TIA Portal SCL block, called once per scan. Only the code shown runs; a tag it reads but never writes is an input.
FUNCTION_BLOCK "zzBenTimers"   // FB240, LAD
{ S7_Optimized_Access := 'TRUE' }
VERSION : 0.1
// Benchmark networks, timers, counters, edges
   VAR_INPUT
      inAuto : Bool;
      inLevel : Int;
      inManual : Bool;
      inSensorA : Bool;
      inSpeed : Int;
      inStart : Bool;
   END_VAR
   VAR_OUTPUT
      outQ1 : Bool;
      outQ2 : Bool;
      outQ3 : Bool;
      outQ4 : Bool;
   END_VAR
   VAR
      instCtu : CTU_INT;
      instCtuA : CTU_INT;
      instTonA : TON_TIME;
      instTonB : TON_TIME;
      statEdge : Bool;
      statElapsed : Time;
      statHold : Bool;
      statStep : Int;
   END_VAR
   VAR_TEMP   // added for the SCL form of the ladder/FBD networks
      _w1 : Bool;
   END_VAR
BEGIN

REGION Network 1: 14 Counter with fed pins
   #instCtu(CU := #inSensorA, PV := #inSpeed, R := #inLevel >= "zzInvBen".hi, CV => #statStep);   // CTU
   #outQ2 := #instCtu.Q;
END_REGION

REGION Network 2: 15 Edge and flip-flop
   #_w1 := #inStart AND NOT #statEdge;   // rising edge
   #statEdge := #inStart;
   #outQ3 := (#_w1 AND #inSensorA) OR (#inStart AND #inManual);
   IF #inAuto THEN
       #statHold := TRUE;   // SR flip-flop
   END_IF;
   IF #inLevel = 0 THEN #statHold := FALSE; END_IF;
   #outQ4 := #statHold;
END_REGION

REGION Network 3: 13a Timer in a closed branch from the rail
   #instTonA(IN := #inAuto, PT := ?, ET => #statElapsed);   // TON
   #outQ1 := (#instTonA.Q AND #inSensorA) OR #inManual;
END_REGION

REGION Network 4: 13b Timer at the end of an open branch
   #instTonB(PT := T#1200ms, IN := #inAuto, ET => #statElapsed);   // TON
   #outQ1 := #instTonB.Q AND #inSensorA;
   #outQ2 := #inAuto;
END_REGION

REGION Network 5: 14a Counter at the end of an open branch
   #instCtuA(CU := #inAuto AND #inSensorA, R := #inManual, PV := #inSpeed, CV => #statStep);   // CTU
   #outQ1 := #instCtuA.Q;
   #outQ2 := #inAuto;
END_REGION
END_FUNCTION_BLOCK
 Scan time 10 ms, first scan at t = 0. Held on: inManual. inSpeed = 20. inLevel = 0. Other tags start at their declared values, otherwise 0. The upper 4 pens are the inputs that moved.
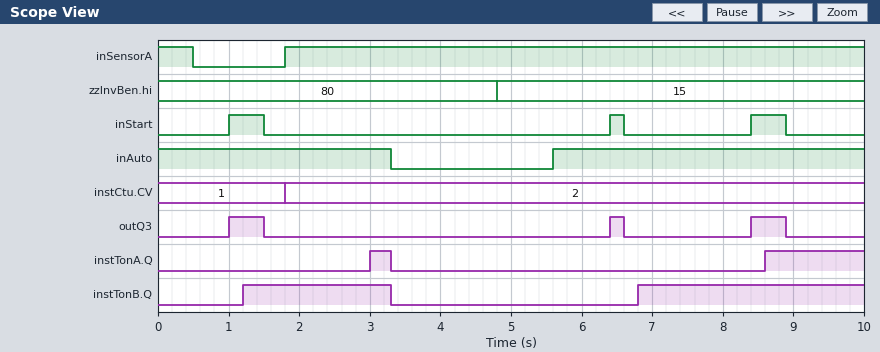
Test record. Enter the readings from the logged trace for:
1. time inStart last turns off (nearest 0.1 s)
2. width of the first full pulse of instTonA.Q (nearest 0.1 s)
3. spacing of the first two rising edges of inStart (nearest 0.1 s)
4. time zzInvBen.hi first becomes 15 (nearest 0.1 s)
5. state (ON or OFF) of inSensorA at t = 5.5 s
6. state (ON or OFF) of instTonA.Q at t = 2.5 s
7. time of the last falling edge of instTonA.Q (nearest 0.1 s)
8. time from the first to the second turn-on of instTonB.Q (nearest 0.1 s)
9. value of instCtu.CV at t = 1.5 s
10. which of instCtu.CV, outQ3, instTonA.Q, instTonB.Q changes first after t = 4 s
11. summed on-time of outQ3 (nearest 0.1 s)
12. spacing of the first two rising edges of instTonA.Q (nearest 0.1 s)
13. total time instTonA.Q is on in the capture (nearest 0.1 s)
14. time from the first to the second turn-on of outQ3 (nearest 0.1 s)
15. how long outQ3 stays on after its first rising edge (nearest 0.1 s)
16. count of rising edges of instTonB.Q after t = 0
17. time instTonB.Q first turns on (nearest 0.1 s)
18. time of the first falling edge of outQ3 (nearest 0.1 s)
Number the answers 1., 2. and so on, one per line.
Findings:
1. 8.9 s
2. 0.3 s
3. 5.4 s
4. 4.8 s
5. ON
6. OFF
7. 3.3 s
8. 5.6 s
9. 1
10. outQ3
11. 1.2 s
12. 5.6 s
13. 1.7 s
14. 5.4 s
15. 0.5 s
16. 2
17. 1.2 s
18. 1.5 s
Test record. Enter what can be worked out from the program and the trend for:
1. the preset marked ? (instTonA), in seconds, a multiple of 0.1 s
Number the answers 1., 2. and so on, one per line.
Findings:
1. 3.0 s
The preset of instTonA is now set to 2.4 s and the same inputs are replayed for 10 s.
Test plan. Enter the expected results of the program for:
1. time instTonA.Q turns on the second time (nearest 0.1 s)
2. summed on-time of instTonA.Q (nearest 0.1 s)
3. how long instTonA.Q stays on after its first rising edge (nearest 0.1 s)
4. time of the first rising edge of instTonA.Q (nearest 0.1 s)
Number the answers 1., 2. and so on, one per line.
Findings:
1. 8.0 s
2. 2.9 s
3. 0.9 s
4. 2.4 s
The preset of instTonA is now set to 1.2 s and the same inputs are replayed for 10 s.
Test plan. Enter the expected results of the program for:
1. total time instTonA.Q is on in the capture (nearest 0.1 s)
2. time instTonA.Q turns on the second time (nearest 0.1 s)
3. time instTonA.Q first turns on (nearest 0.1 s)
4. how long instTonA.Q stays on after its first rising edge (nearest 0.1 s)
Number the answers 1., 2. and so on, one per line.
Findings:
1. 5.3 s
2. 6.8 s
3. 1.2 s
4. 2.1 s
